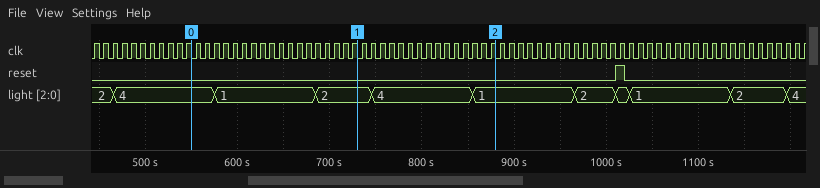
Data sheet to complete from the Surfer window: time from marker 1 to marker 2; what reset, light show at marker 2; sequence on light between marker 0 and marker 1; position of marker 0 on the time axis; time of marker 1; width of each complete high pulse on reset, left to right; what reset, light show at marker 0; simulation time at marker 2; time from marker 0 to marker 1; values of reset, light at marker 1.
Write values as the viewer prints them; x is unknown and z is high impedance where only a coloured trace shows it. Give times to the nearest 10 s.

150 s
reset=0, light=1
4, 1, 2
550 s
730 s
10 s
reset=0, light=4
880 s
180 s
reset=0, light=2
